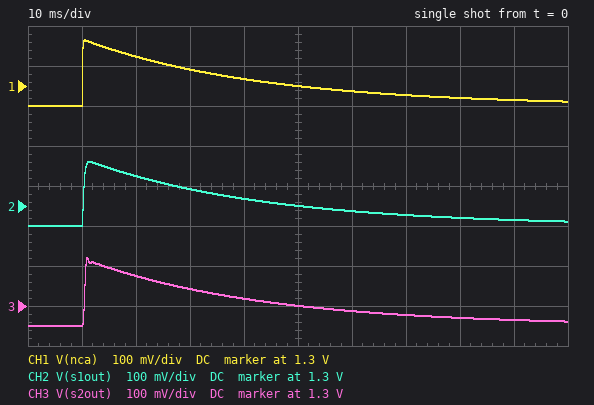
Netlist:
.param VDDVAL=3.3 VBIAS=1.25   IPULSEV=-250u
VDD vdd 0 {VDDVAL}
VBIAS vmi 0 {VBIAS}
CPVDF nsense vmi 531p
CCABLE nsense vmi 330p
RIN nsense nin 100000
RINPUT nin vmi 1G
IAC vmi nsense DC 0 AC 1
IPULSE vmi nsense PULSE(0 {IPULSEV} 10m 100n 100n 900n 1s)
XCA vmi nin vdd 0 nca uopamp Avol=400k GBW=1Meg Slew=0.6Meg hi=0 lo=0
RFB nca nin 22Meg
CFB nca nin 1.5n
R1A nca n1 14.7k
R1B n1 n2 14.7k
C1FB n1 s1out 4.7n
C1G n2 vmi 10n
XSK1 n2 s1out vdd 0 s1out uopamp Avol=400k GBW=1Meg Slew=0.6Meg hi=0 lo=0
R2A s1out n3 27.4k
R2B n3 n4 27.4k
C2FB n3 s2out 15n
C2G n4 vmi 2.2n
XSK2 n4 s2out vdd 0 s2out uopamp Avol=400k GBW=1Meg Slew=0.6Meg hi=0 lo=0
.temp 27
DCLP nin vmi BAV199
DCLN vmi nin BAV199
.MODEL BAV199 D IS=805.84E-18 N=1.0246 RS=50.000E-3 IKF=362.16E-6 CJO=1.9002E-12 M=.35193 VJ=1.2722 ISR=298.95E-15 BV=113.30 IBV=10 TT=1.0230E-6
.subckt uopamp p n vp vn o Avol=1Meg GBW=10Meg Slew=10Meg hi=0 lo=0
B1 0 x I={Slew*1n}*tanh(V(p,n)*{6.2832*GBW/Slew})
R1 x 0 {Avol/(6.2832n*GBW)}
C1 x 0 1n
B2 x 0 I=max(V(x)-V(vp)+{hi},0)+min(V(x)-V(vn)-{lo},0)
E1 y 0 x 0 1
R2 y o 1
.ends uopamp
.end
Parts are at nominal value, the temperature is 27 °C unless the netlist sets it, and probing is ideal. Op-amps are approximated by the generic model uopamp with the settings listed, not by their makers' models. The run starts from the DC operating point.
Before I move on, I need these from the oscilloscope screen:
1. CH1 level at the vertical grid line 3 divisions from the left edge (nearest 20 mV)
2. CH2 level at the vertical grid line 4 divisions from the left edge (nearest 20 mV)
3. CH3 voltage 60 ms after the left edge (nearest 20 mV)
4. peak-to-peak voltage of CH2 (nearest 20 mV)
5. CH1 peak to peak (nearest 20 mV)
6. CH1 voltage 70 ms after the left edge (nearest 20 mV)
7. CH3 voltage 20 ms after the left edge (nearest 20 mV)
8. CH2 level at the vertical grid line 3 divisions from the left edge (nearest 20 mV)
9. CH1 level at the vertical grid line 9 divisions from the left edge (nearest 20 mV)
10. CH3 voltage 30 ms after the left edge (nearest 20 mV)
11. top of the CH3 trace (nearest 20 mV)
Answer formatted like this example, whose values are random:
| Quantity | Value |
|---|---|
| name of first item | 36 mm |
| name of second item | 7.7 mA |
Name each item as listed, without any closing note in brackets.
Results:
| Quantity | Value |
|---|---|
| CH1 level at the vertical grid line 3 divisions from the left edge | 1.34 V |
| CH2 level at the vertical grid line 4 divisions from the left edge | 1.32 V |
| CH3 voltage 60 ms after the left edge | 1.28 V |
| peak-to-peak voltage of CH2 | 160 mV |
| CH1 peak to peak | 160 mV |
| CH1 voltage 70 ms after the left edge | 1.28 V |
| CH3 voltage 20 ms after the left edge | 1.38 V |
| CH2 level at the vertical grid line 3 divisions from the left edge | 1.34 V |
| CH1 level at the vertical grid line 9 divisions from the left edge | 1.26 V |
| CH3 voltage 30 ms after the left edge | 1.34 V |
| top of the CH3 trace | 1.42 V |
